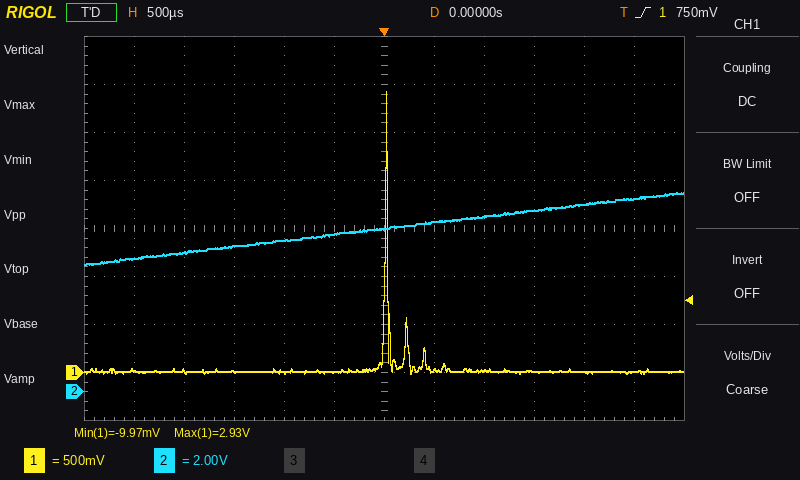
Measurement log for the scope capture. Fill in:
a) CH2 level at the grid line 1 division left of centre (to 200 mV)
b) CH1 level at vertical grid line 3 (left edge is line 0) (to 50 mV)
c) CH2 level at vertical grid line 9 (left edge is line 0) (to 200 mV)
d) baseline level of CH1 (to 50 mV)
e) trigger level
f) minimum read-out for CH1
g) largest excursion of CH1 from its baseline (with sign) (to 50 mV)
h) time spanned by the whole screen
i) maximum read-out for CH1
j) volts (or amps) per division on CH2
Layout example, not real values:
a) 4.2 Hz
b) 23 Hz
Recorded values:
a) 6.6 V
b) 0 mV
c) 7.6 V
d) 0 mV
e) 750 mV
f) -9.97 mV
g) +2.90 V
h) 6 ms
i) 2.93 V
j) 2 V
